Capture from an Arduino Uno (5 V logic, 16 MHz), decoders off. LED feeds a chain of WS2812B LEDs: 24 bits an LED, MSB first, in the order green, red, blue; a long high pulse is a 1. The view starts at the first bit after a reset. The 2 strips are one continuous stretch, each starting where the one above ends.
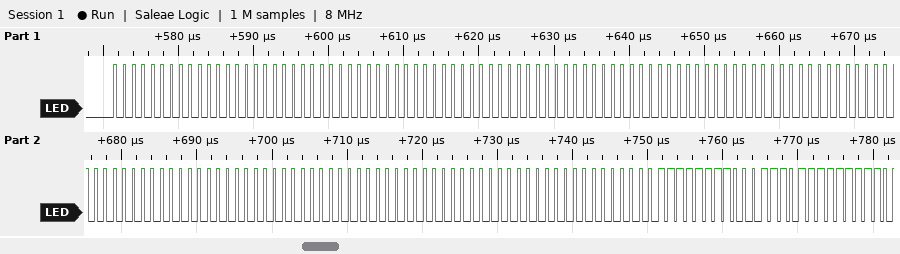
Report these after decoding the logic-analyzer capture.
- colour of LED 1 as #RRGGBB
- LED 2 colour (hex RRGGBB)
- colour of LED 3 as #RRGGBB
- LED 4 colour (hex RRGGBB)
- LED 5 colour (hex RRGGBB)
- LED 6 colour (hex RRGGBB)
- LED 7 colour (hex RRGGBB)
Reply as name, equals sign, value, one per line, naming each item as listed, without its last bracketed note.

colour of LED 1 as #RRGGBB = #000000
LED 2 colour = #000000
colour of LED 3 as #RRGGBB = #000000
LED 4 colour = #000000
LED 5 colour = #000000
LED 6 colour = #000000
LED 7 colour = #1DFFFF
